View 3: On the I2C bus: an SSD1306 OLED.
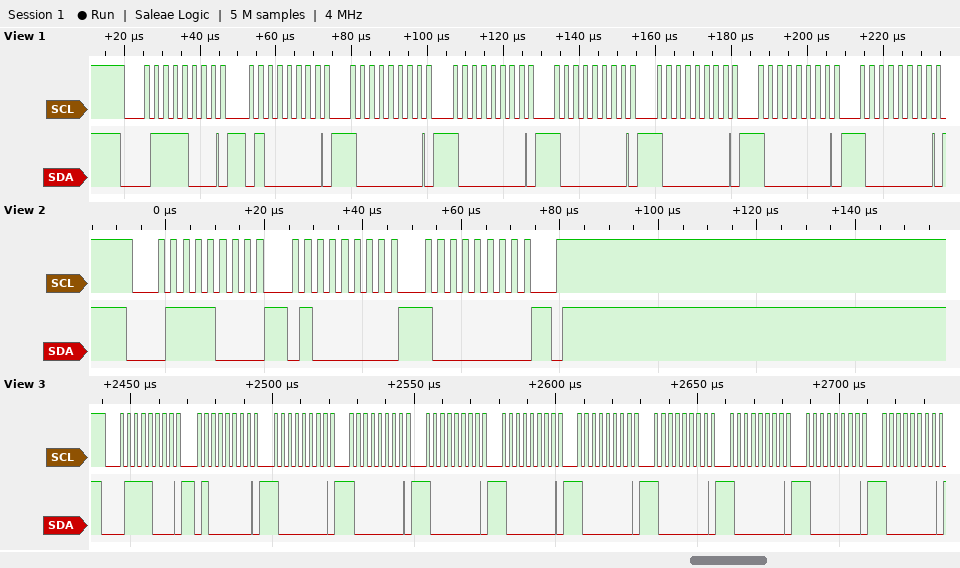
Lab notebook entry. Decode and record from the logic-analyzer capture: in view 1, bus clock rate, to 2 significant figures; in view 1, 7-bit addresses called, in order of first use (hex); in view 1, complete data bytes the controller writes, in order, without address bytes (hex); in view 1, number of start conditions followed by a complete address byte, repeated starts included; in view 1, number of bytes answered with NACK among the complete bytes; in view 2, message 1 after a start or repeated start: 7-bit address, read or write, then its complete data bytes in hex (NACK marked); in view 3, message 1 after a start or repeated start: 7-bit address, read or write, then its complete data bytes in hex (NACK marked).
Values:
400 kHz
0x3C
40 80 80 80 80 80 80
1
0
0x3C write: 40 80
0x3C write: 40 80 80 80 80 80 80 80 80 80
